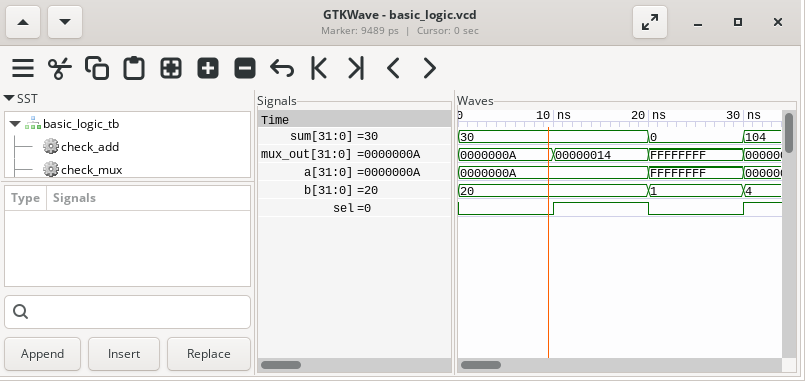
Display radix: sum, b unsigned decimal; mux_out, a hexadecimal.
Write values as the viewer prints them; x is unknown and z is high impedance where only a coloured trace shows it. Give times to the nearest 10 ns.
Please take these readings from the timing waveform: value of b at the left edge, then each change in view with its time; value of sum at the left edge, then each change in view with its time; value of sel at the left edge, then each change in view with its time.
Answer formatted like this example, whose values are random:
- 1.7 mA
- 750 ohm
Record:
- 20, 1 at 20 ns, 4 at 30 ns
- 30, 0 at 20 ns, 104 at 30 ns
- 0, 1 at 10 ns, 0 at 20 ns, 1 at 30 ns
